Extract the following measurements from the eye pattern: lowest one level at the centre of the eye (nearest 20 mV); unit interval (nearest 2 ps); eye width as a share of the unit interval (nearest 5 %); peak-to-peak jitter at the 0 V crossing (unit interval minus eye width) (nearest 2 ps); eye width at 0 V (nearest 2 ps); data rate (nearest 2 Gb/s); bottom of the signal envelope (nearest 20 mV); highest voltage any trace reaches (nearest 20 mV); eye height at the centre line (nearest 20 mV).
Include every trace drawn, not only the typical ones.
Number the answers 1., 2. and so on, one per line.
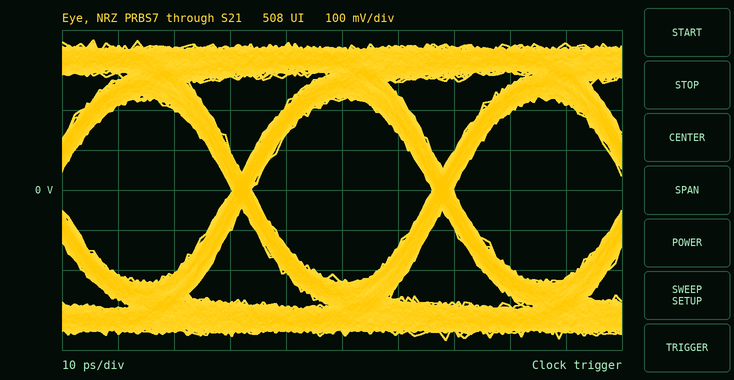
1. 220 mV
2. 36 ps
3. 90 %
4. 4 ps
5. 32 ps
6. 28 Gb/s
7. -380 mV
8. 380 mV
9. 460 mV
